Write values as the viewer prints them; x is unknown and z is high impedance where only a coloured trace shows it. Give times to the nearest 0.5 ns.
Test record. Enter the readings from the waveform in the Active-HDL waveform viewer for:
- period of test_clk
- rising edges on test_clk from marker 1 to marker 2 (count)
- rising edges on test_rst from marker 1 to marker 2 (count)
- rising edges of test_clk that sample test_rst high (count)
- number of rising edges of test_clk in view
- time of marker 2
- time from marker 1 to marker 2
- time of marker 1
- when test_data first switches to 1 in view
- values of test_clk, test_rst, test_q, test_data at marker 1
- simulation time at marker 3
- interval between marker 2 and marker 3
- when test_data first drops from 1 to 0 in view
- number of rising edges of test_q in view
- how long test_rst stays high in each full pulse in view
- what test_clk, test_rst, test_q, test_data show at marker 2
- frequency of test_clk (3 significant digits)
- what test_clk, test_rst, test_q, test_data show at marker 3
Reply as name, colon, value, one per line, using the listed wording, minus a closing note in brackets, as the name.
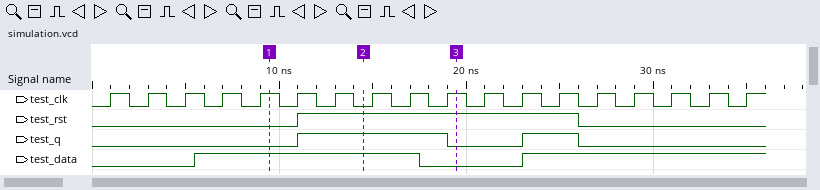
period of test_clk: 2 ns
rising edges on test_clk from marker 1 to marker 2: 2
rising edges on test_rst from marker 1 to marker 2: 1
rising edges of test_clk that sample test_rst high: 7
number of rising edges of test_clk in view: 18
time of marker 2: 14.5 ns
time from marker 1 to marker 2: 5 ns
time of marker 1: 9.5 ns
when test_data first switches to 1 in view: 5.5 ns
values of test_clk, test_rst, test_q, test_data at marker 1: test_clk=1, test_rst=0, test_q=0, test_data=1
simulation time at marker 3: 19.5 ns
interval between marker 2 and marker 3: 5 ns
when test_data first drops from 1 to 0 in view: 17.5 ns
number of rising edges of test_q in view: 2
how long test_rst stays high in each full pulse in view: 15 ns
what test_clk, test_rst, test_q, test_data show at marker 2: test_clk=0, test_rst=1, test_q=1, test_data=1
frequency of test_clk: 500 MHz
what test_clk, test_rst, test_q, test_data show at marker 3: test_clk=1, test_rst=1, test_q=0, test_data=0
